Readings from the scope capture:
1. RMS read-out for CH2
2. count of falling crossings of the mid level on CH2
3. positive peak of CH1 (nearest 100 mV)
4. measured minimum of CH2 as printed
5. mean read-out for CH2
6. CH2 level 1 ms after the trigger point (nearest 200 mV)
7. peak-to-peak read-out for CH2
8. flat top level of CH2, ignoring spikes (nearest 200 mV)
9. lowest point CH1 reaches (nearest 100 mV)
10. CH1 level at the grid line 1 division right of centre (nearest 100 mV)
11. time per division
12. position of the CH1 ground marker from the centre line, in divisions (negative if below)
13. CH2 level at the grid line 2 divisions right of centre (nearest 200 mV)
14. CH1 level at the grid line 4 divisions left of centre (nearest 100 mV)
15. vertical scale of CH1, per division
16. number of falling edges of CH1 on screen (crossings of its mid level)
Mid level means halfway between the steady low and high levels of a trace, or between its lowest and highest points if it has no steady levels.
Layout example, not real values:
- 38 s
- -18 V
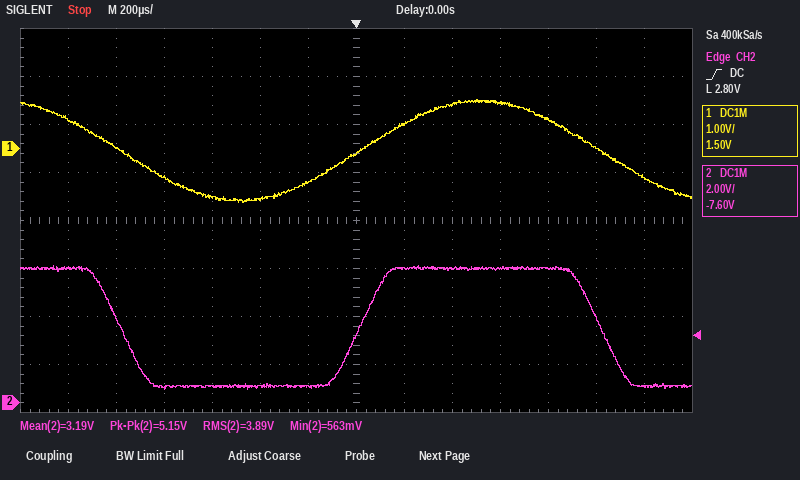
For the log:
- 3.89 V
- 2
- 1.0 V
- 563 mV
- 3.19 V
- 3.6 V
- 5.15 V
- 5.6 V
- -1.1 V
- 500 mV
- 200 µs
- +1.5 div
- 5.6 V
- -600 mV
- 1 V
- 2
